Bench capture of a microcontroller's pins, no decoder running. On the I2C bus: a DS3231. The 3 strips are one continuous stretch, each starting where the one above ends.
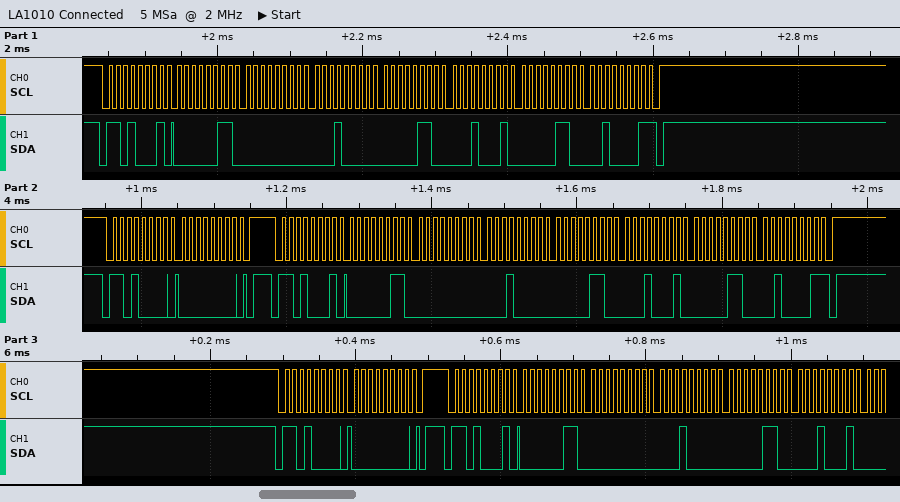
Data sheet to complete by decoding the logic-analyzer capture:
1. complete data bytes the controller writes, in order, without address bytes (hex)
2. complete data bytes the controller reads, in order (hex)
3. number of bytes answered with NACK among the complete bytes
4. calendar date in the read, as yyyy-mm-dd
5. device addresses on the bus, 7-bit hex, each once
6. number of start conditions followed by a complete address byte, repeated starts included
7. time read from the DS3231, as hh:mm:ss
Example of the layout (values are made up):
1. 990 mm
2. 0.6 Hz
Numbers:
1. 00 00
2. 03 00 10 06 11 06 21 03 00 10 06 11 06 21 03 00 10 06 11
3. 2
4. 2021-06-11
5. 0x68
6. 5
7. 10:00:03
